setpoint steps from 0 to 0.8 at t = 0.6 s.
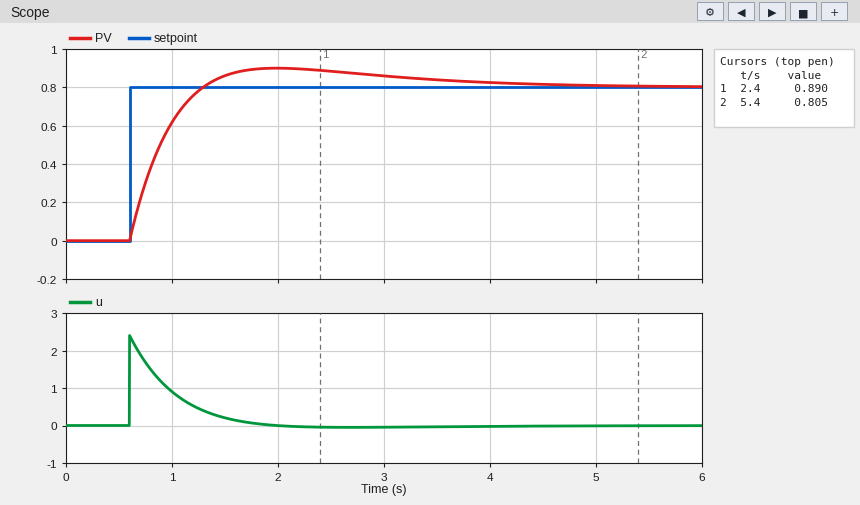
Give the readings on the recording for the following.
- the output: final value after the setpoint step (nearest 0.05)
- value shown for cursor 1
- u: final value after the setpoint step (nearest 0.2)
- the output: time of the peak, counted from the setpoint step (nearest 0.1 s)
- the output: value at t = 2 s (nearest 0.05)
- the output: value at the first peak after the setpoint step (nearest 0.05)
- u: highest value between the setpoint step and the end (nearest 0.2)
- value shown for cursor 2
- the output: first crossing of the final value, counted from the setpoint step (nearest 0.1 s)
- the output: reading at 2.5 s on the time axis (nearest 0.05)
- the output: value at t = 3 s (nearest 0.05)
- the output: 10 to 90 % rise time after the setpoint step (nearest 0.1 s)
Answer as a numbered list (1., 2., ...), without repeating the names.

1. 0.80
2. 0.890
3. 0.0
4. 1.4 s
5. 0.90
6. 0.90
7. 2.4
8. 0.805
9. 0.7 s
10. 0.90
11. 0.85
12. 0.5 s
